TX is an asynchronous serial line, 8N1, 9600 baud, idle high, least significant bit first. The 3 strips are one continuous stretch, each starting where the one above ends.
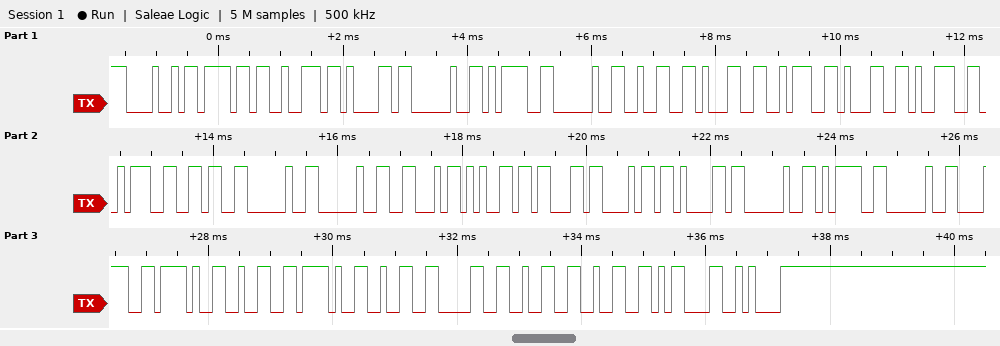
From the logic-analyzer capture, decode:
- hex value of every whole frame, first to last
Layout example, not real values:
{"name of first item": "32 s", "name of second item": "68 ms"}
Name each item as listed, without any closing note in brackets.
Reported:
{"hex value of every whole frame, first to last": "0x48 0x6F 0x72 0x61 0x20 0x3D 0x20 0x32 0x31 0x3A 0x31 0x39 0x3A 0x36 0x20 0x20 0x46 0x65 0x63 0x68 0x61 0x20 0x3D 0x20 0x38 0x2F 0x32 0x2F 0x32 0x30 0x32 0x32 0x0D 0x0A"}
